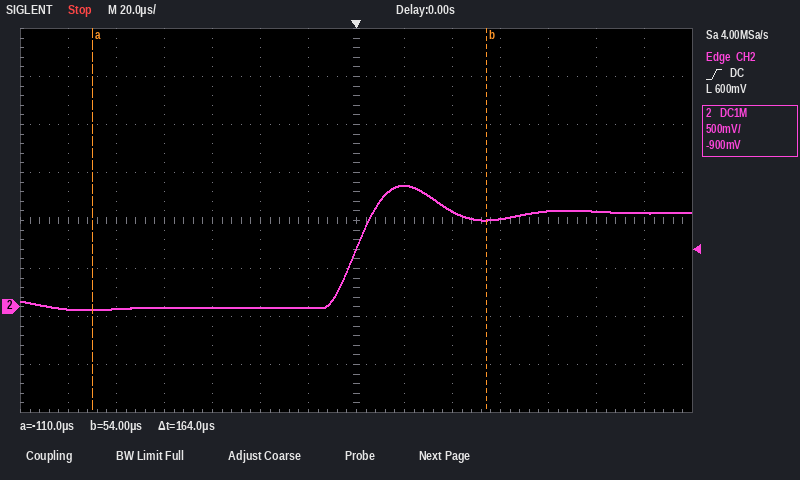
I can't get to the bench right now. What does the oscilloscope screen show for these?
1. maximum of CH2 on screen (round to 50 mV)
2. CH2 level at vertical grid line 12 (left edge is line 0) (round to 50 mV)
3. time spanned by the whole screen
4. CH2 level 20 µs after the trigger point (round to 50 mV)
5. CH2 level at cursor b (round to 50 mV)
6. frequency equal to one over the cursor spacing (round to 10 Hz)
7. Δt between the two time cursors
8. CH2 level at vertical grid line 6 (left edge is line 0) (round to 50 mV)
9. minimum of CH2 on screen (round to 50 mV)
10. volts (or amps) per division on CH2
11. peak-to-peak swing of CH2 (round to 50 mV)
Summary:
1.25 V
1.00 V
280 µs
1.25 V
900 mV
6.10 kHz
164 µs
0 mV
-50 mV
500 mV
1.30 V
